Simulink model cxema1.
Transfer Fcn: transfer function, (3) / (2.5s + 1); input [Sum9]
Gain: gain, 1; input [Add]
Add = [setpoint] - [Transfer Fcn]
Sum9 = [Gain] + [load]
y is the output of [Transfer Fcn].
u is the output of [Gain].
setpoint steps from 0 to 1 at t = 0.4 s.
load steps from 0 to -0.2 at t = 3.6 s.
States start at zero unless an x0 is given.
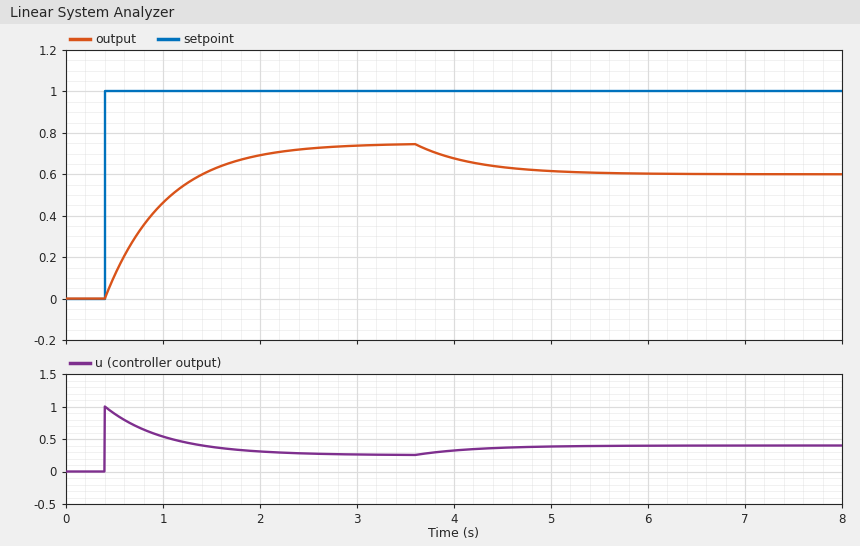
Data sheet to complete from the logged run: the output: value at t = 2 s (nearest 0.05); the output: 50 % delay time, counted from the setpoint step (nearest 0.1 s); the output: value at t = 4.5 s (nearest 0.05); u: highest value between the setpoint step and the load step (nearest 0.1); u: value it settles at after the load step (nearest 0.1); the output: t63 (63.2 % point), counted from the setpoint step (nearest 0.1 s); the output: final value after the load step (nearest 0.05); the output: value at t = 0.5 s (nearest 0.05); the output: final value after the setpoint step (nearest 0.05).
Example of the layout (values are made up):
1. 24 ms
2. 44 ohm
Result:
1. 0.70
2. 0.4 s
3. 0.65
4. 1.0
5. 0.4
6. 0.6 s
7. 0.60
8. 0.10
9. 0.75
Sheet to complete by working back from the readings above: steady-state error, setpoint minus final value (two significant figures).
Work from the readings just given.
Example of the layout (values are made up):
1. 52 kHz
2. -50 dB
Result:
1. 0.25
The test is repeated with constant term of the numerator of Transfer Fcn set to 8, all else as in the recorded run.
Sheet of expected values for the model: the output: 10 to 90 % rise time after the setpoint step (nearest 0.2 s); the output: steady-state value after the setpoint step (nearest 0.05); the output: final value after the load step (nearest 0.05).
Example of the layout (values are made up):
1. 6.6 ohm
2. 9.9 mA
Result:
1. 0.6 s
2. 0.90
3. 0.70
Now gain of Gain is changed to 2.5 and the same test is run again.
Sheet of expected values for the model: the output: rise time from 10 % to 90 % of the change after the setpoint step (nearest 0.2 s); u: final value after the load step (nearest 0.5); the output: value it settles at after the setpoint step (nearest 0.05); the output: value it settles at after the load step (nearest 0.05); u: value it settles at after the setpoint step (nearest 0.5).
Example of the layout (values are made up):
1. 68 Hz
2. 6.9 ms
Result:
1. 0.6 s
2. 0.5
3. 0.90
4. 0.80
5. 0.5
